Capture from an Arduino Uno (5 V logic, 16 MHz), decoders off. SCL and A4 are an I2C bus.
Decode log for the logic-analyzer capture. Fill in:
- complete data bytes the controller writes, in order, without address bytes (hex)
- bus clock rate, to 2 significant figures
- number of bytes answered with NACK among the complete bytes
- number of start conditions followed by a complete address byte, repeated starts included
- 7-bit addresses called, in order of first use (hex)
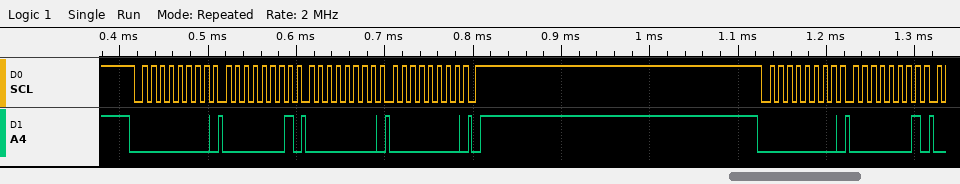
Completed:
01 00 00 01
100 kHz
0
2
0x00
